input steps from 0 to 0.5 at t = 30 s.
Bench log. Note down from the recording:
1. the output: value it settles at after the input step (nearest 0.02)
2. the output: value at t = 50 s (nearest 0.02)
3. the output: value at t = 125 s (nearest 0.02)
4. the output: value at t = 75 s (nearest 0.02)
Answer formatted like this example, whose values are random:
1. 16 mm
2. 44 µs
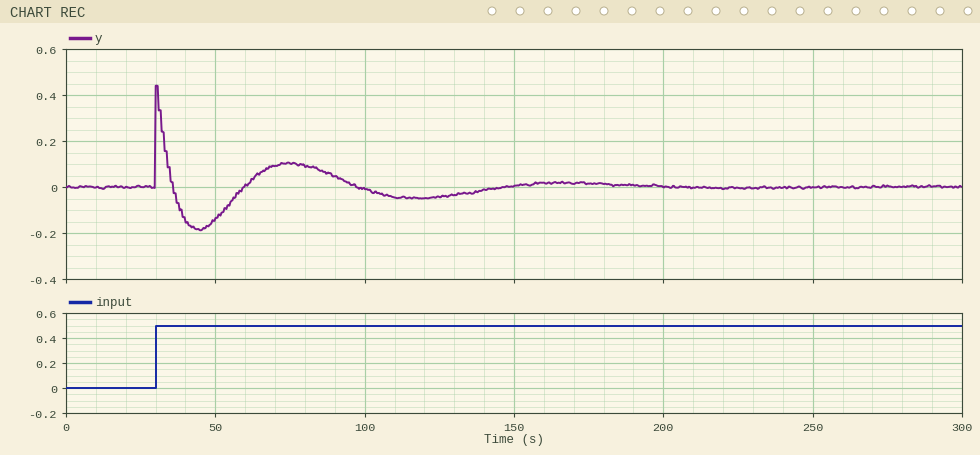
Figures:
1. 0.00
2. -0.14
3. -0.04
4. 0.10
